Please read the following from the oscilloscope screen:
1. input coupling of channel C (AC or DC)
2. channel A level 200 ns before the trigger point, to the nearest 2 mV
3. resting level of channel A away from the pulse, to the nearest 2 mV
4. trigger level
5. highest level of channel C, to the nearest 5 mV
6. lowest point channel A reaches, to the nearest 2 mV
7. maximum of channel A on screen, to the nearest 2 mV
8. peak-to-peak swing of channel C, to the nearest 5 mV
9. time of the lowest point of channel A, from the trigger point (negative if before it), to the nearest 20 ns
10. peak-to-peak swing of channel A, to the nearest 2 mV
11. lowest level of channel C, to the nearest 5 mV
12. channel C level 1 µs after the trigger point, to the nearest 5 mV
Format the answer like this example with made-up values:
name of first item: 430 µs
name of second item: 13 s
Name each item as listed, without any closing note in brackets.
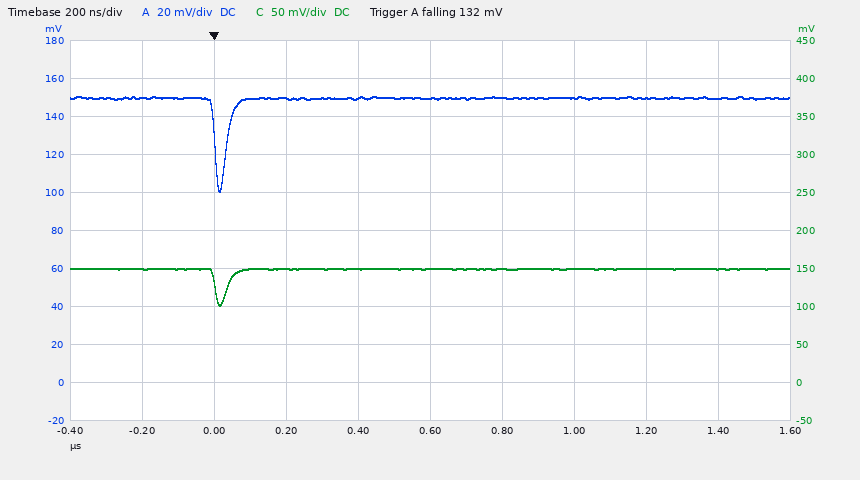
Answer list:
input coupling of channel C: DC
channel A level 200 ns before the trigger point, to the nearest 2 mV: 150 mV
resting level of channel A away from the pulse, to the nearest 2 mV: 150 mV
trigger level: 132 mV
highest level of channel C, to the nearest 5 mV: 150 mV
lowest point channel A reaches, to the nearest 2 mV: 100 mV
maximum of channel A on screen, to the nearest 2 mV: 150 mV
peak-to-peak swing of channel C, to the nearest 5 mV: 50 mV
time of the lowest point of channel A, from the trigger point (negative if before it), to the nearest 20 ns: +20 ns
peak-to-peak swing of channel A, to the nearest 2 mV: 50 mV
lowest level of channel C, to the nearest 5 mV: 100 mV
channel C level 1 µs after the trigger point, to the nearest 5 mV: 150 mV
